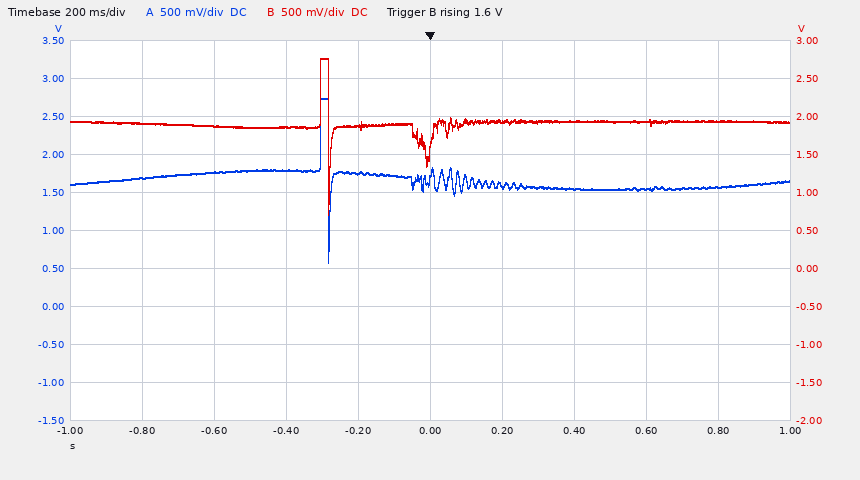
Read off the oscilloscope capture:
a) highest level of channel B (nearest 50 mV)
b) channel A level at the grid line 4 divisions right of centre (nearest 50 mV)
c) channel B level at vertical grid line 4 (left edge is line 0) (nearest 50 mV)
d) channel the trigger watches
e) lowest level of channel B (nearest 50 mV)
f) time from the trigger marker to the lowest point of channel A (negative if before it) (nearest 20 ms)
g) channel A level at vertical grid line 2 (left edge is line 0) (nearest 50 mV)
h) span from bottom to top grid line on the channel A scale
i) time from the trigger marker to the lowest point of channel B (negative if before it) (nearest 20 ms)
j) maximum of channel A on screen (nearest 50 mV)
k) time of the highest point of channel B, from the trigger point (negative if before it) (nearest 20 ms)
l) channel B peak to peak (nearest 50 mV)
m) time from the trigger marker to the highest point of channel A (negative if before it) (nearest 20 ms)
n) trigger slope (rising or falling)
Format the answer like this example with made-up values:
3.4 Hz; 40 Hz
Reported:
2.75 V; 1.55 V; 1.85 V; channel B; 700 mV; -280 ms; 1.75 V; 5 V; -280 ms; 2.75 V; -300 ms; 2.05 V; -300 ms; rising
